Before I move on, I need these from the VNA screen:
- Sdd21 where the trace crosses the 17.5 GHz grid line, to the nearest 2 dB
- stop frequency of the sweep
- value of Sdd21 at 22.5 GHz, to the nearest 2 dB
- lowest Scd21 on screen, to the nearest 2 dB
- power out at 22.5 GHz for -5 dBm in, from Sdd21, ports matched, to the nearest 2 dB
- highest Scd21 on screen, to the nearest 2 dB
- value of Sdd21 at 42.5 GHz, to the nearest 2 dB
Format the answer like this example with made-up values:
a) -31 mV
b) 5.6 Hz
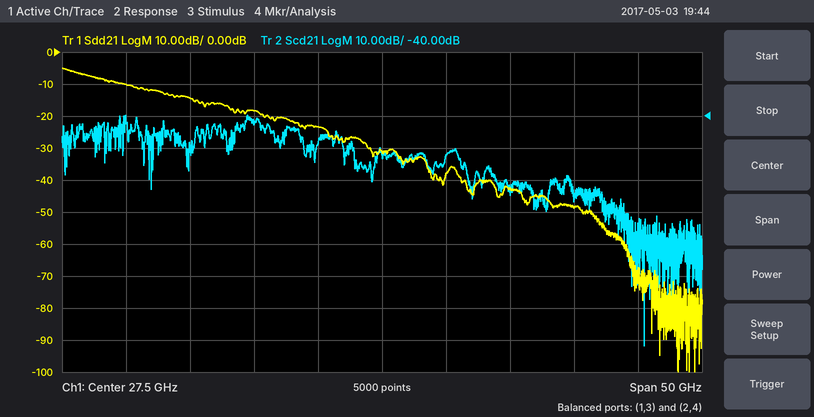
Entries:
a) -18 dB
b) 52.5 GHz
c) -24 dB
d) -112 dB
e) -28 dBm
f) -40 dB
g) -48 dB
